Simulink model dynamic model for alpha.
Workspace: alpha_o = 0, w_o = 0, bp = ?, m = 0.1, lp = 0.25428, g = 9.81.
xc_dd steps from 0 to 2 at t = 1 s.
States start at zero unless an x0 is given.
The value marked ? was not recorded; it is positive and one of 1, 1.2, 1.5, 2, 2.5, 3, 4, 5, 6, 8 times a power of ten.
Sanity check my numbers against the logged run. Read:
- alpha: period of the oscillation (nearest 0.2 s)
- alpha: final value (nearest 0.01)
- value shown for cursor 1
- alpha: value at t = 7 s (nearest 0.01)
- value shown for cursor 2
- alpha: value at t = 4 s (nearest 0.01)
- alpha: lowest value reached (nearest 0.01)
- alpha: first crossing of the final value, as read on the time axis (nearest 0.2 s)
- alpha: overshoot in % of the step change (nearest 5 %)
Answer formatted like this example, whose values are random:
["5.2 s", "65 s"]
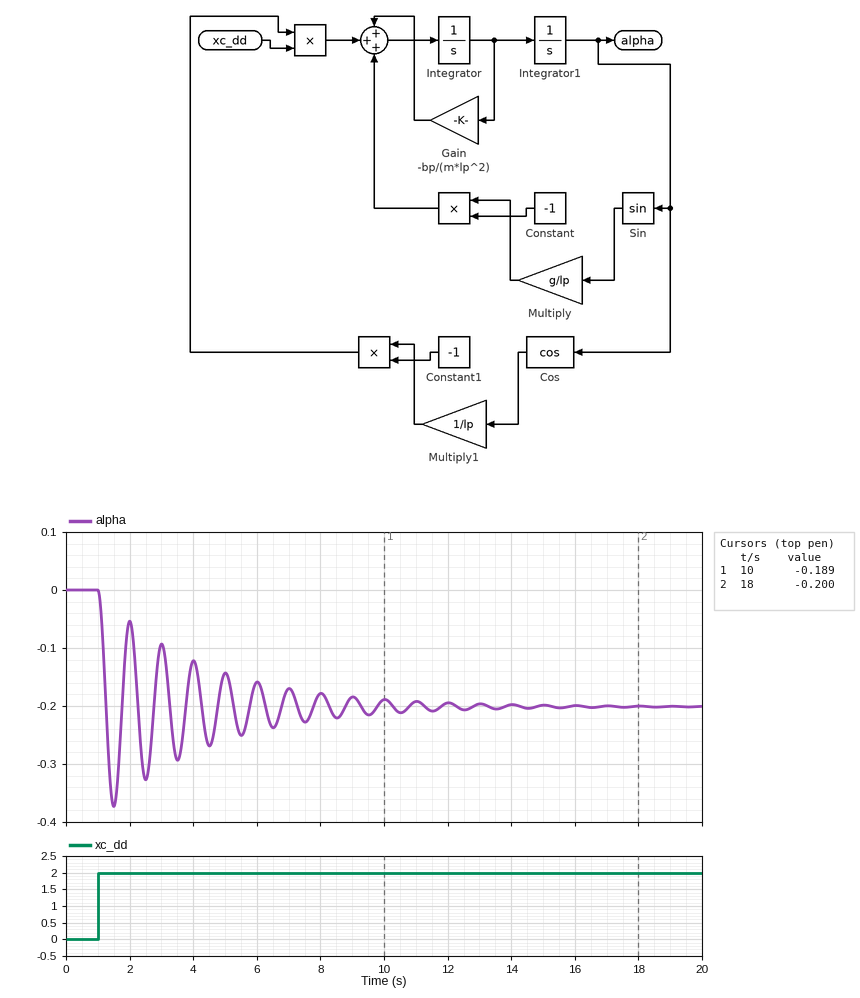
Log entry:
["1.0 s", "-0.20", "-0.189", "-0.17", "-0.200", "-0.12", "-0.37", "1.2 s", "85 %"]
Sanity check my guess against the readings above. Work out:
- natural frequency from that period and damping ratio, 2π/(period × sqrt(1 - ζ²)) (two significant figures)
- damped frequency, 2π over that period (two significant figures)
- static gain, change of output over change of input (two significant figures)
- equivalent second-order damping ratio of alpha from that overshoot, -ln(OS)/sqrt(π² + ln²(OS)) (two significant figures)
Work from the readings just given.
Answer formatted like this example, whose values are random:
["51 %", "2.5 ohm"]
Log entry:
["6.3 rad/s", "6.3 rad/s", "-0.10", "0.052"]
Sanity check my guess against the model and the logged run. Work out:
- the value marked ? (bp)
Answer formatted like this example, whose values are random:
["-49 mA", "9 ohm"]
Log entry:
["0.004"]
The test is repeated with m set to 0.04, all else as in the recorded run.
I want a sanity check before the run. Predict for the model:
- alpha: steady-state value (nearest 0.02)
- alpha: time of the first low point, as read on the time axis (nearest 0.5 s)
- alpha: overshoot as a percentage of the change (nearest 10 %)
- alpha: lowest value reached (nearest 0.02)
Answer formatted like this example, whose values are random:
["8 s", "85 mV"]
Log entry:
["-0.20", "1.5 s", "70 %", "-0.34"]
